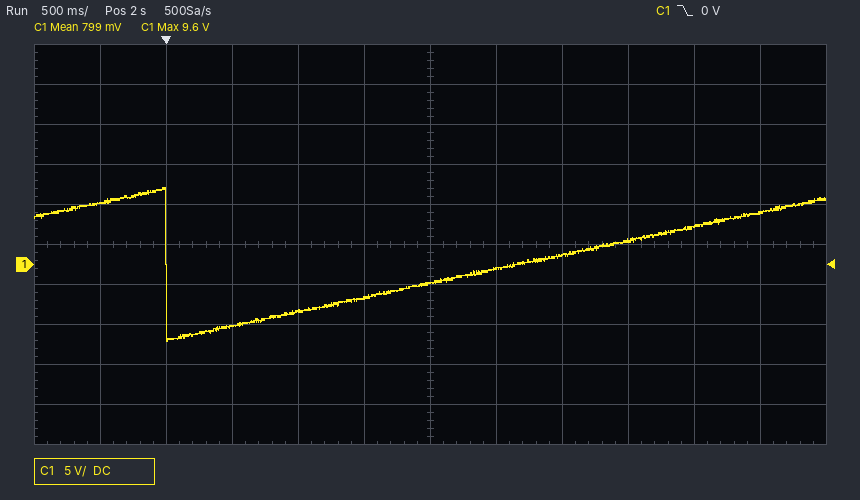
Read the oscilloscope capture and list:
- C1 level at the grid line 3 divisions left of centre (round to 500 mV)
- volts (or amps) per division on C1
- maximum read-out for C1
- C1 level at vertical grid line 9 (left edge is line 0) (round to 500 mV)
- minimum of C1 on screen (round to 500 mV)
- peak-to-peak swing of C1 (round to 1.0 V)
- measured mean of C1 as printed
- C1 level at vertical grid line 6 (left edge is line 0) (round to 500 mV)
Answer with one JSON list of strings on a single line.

["-8.0 V", "5 V", "9.6 V", "3.0 V", "-9.5 V", "19.0 V", "799 mV", "-2.5 V"]
